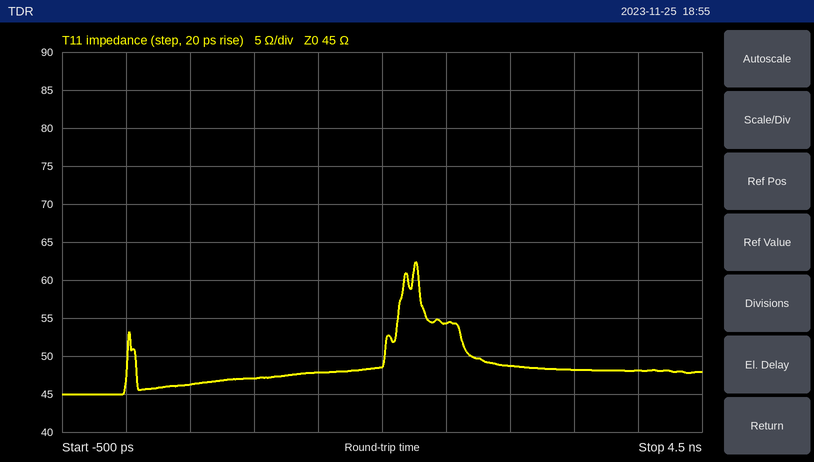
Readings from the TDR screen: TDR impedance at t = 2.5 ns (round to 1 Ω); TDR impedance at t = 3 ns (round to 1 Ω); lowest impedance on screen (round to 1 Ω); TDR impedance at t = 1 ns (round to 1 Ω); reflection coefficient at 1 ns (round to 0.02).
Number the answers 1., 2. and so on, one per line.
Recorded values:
1. 54 Ω
2. 49 Ω
3. 45 Ω
4. 47 Ω
5. +0.02
